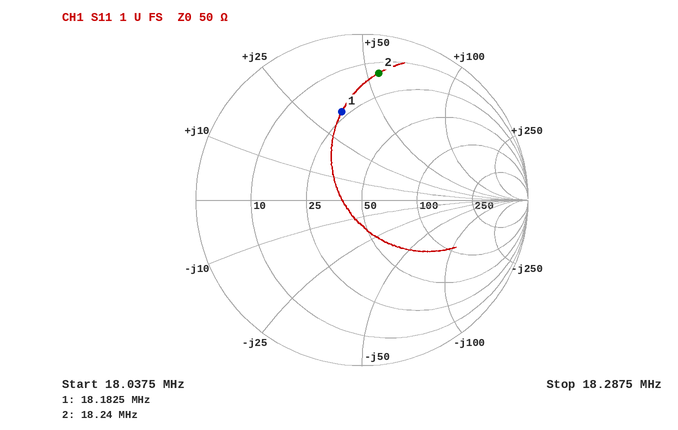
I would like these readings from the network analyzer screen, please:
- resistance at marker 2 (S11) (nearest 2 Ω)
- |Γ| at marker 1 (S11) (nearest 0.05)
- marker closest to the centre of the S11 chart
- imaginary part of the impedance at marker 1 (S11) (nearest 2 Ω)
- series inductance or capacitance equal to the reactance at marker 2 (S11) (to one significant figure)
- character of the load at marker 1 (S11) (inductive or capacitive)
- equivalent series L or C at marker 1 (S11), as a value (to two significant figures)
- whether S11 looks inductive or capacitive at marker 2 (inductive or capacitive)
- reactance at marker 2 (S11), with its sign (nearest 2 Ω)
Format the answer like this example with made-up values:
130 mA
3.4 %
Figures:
14 Ω
0.55
marker 1
+34 Ω
500 nH
inductive
300 nH
inductive
+54 Ω
